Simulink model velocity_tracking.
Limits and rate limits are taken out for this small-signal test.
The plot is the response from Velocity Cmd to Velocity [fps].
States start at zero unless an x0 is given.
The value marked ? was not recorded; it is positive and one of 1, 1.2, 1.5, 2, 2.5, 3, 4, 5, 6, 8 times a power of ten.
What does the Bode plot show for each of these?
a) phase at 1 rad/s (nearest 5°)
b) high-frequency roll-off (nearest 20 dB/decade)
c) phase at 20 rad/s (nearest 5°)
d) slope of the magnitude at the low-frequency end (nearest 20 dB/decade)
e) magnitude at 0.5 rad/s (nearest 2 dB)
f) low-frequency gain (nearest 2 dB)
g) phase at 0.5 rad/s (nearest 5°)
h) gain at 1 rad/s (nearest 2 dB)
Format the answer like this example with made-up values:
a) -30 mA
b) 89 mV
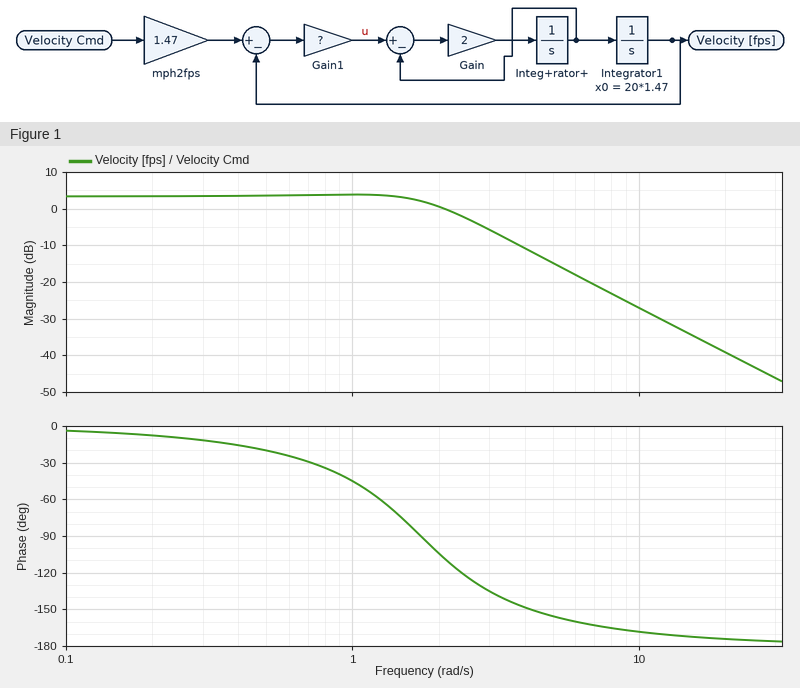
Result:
a) -45°
b) -40 dB/decade
c) -175°
d) 0 dB/decade
e) 4 dB
f) 4 dB
g) -20°
h) 4 dB
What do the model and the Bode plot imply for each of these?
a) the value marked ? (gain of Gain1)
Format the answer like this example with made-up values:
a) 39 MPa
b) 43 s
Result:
a) 1.5
